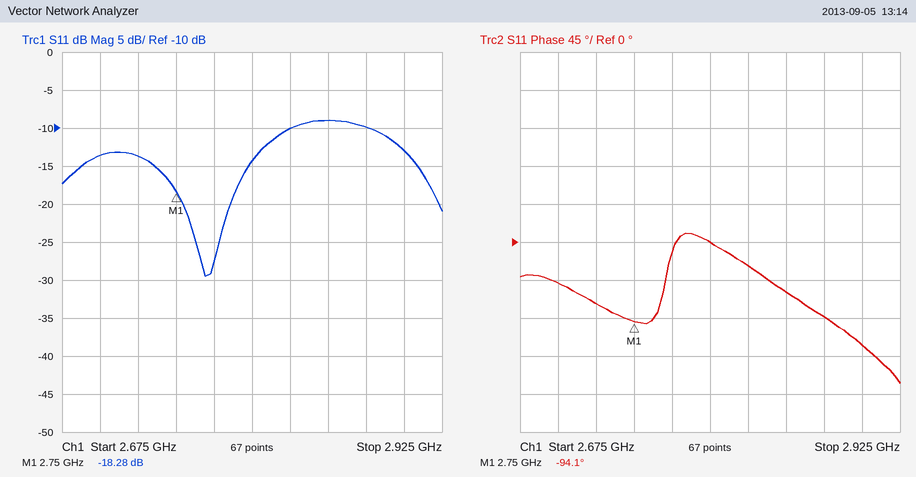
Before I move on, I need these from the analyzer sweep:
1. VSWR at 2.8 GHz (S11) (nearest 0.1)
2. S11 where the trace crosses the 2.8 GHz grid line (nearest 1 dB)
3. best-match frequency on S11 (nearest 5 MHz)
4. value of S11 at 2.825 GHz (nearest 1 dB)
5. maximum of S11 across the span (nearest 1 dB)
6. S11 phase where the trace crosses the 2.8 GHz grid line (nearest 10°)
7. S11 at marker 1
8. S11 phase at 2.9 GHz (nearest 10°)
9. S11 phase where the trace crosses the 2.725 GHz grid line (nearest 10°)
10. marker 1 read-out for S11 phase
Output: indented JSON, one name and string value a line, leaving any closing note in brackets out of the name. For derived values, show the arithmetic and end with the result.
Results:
{
  "VSWR at 2.8 GHz (S11)": "|Γ| = 10^(-14/20) = 0.1995; VSWR = (1 + 0.1995)/(1 − 0.1995) ≈ 1.5",
  "S11 where the trace crosses the 2.8 GHz grid line": "-14 dB",
  "best-match frequency on S11": "2.770 GHz",
  "value of S11 at 2.825 GHz": "-10 dB",
  "maximum of S11 across the span": "-9 dB",
  "S11 phase where the trace crosses the 2.8 GHz grid line": "0°",
  "S11 at marker 1": "-18.28 dB",
  "S11 phase at 2.9 GHz": "-120°",
  "S11 phase where the trace crosses the 2.725 GHz grid line": "-70°",
  "marker 1 read-out for S11 phase": "-94.1°"
}
